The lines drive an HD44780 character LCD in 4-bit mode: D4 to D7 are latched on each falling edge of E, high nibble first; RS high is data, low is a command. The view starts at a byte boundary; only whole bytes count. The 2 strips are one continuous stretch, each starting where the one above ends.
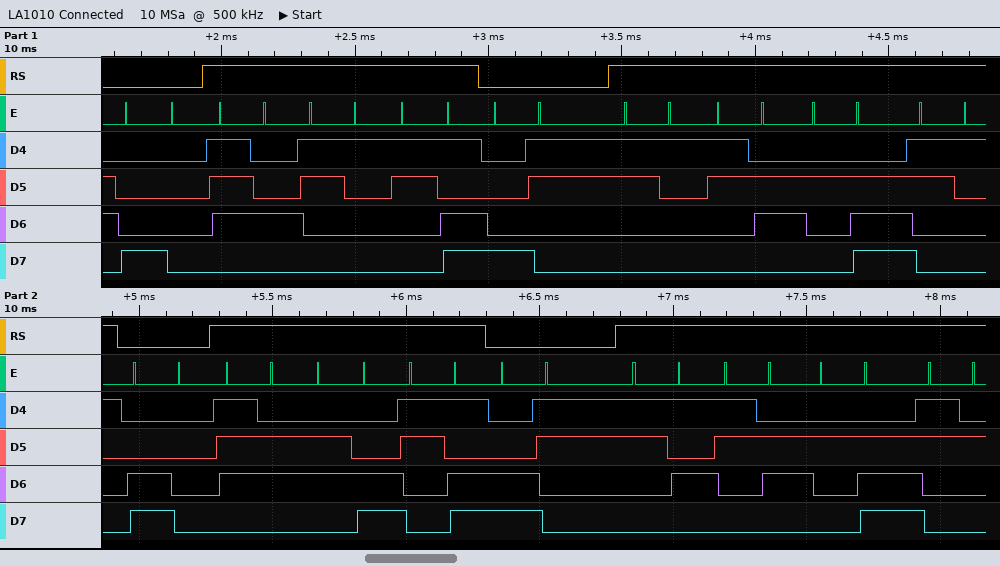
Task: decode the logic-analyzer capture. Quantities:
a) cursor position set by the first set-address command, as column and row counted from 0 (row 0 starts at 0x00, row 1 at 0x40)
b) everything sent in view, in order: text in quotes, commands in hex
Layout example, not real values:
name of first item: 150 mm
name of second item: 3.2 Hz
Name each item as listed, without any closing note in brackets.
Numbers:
cursor position set by the first set-address command, as column and row counted from 0: column 0, row 0
everything sent in view, in order: text in quotes, commands in hex: 0x80 "t1=" 0x83 "16.1" 0xC0 "vl=" 0xC3 "56.2"
